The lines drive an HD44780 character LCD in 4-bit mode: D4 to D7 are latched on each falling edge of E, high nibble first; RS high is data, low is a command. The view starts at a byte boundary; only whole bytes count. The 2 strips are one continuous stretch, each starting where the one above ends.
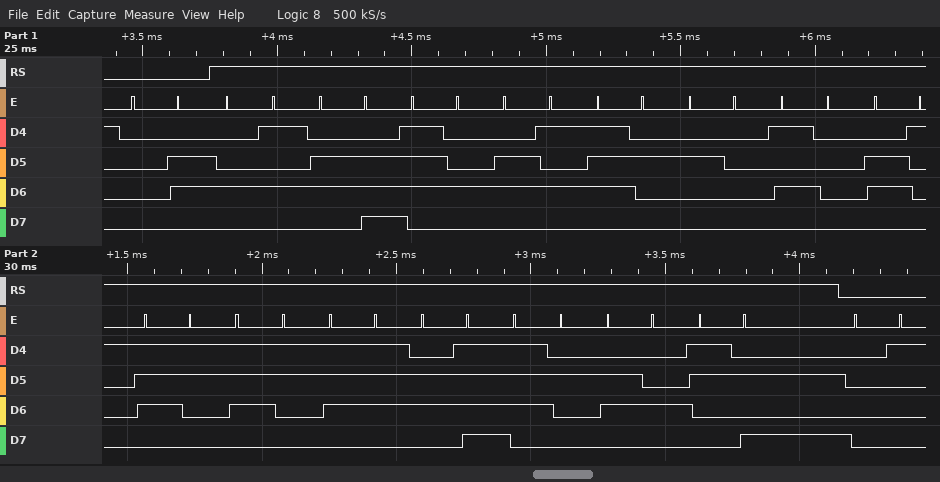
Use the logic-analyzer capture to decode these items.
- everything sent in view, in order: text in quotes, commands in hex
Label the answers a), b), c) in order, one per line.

a) 0x06 "Enter Password:" 0x01
